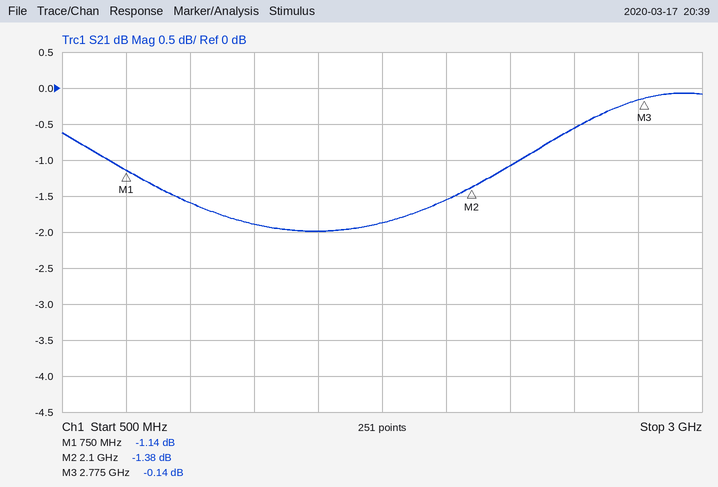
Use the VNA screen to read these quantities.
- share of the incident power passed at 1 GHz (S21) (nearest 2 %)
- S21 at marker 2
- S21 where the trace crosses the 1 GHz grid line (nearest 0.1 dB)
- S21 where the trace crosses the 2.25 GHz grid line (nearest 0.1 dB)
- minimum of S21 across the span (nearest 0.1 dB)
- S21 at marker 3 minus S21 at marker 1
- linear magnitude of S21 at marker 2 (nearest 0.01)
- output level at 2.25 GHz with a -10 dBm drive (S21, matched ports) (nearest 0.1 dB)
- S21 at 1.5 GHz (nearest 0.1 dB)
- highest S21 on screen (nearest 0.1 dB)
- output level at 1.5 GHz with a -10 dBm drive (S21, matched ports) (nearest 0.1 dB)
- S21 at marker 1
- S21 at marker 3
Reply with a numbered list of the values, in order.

1. 70 %
2. -1.38 dB
3. -1.6 dB
4. -1.1 dB
5. -2.0 dB
6. 1.00 dB
7. 0.85
8. -11.1 dBm
9. -2.0 dB
10. -0.1 dB
11. -12.0 dBm
12. -1.14 dB
13. -0.14 dB
